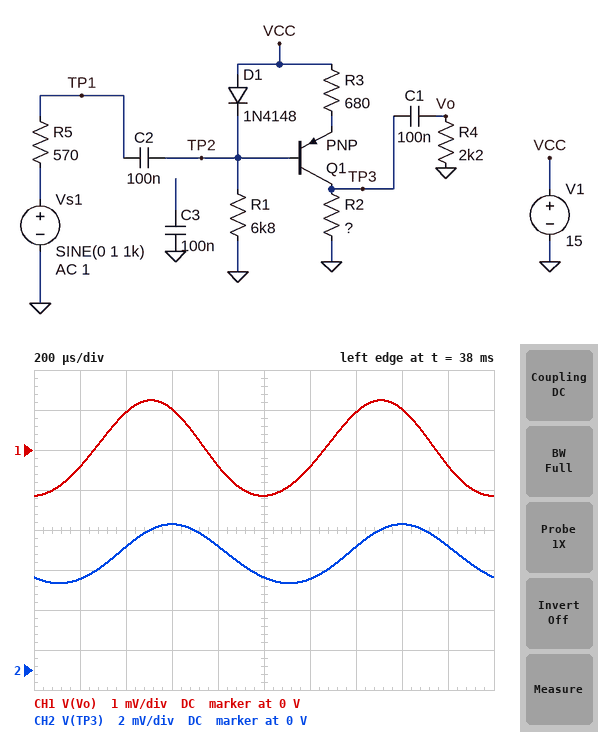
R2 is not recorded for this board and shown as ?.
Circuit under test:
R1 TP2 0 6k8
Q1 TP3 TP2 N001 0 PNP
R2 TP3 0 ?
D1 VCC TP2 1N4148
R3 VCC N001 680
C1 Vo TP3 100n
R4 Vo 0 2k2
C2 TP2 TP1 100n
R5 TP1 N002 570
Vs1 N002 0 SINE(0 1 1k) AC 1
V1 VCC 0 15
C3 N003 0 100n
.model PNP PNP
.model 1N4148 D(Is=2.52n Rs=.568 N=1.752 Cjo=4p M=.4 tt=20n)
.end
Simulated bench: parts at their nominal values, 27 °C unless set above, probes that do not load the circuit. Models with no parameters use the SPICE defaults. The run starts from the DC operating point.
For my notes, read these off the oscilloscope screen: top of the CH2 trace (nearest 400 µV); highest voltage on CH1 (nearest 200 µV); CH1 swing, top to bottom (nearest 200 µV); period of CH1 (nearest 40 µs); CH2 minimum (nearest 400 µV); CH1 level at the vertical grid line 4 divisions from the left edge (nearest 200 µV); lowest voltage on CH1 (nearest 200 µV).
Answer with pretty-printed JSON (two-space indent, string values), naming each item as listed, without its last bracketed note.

{
  "top of the CH2 trace": "7.2 mV",
  "highest voltage on CH1": "1.2 mV",
  "CH1 swing, top to bottom": "2.4 mV",
  "period of CH1": "1.00 ms",
  "CH2 minimum": "4.4 mV",
  "CH1 level at the vertical grid line 4 divisions from the left edge": "-400 µV",
  "lowest voltage on CH1": "-1.2 mV"
}
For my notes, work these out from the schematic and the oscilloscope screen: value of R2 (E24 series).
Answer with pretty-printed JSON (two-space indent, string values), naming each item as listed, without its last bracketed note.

{
  "value of R2": "2.4 kΩ"
}
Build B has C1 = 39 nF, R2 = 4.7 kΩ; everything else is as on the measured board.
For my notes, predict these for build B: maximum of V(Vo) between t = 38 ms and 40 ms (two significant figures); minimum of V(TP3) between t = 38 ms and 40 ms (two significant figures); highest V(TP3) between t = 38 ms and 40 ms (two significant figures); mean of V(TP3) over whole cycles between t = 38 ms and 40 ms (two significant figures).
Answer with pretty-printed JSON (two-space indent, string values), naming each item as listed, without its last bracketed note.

{
  "maximum of V(Vo) between t = 38 ms and 40 ms": "1.5 mV",
  "minimum of V(TP3) between t = 38 ms and 40 ms": "8.4 mV",
  "highest V(TP3) between t = 38 ms and 40 ms": "14 mV",
  "mean of V(TP3) over whole cycles between t = 38 ms and 40 ms": "11 mV"
}
